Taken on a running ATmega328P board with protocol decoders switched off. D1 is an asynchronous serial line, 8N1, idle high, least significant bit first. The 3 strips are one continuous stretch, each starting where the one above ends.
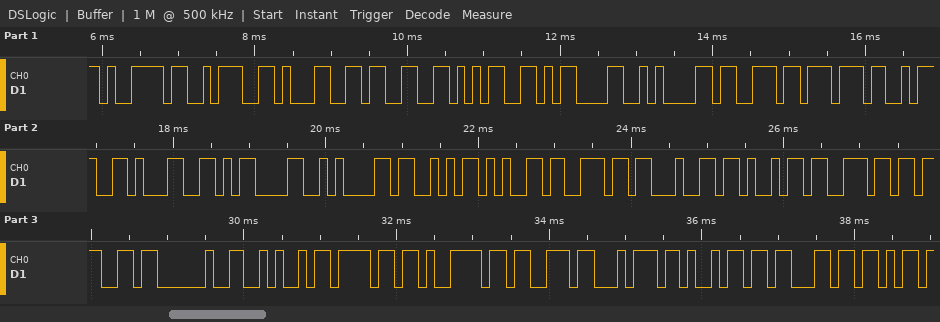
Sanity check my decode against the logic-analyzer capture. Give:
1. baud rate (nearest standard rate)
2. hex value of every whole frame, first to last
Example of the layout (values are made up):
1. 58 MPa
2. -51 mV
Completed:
1. 9600 baud
2. 79 3A 31 33 35 0D 0A 73 77 3A 31 0D 0A 53 65 6E 64 69 6E 67 20 4A 6F 79 73 74 69 63 6B
